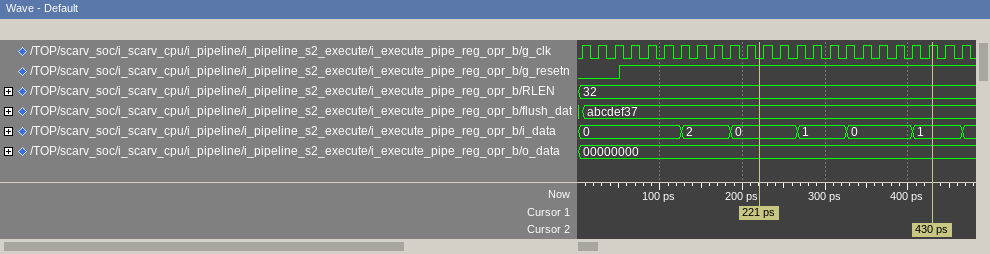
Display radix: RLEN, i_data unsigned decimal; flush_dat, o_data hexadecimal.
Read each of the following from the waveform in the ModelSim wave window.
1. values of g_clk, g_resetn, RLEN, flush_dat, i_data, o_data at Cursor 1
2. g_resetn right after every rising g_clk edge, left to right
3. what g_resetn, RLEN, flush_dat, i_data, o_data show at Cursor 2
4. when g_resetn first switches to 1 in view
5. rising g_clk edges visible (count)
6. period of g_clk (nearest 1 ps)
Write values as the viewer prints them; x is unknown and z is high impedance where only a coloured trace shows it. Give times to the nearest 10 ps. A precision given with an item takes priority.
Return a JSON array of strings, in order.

["g_clk=0, g_resetn=1, RLEN=32, flush_dat=abcdef37, i_data=0, o_data=00000000", "0 0 0 1 1 1 1 1 1 1 1 1 1 1 1 1 1 1 1 1 1 1 1 1", "g_resetn=1, RLEN=32, flush_dat=abcdef37, i_data=1, o_data=00000000", "50 ps", "24", "20 ps"]
